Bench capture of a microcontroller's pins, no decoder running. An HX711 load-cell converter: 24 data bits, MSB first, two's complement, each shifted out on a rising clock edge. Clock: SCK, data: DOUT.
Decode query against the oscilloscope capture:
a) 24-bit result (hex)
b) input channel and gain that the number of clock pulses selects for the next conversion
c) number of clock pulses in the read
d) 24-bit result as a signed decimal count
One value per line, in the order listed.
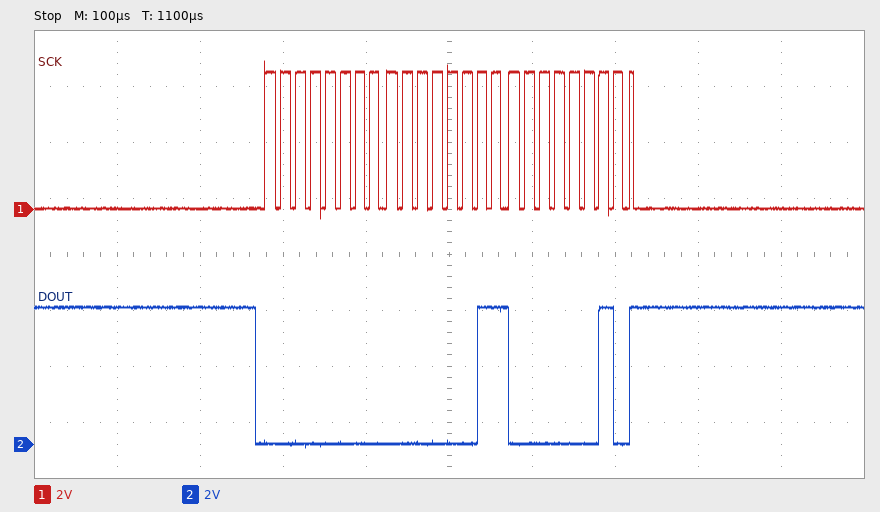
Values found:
0x000302
channel A, gain 128
25
770
